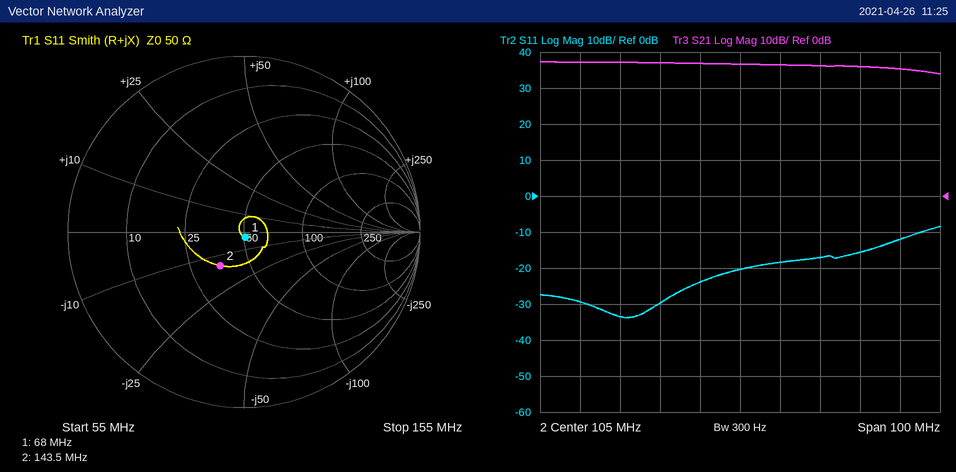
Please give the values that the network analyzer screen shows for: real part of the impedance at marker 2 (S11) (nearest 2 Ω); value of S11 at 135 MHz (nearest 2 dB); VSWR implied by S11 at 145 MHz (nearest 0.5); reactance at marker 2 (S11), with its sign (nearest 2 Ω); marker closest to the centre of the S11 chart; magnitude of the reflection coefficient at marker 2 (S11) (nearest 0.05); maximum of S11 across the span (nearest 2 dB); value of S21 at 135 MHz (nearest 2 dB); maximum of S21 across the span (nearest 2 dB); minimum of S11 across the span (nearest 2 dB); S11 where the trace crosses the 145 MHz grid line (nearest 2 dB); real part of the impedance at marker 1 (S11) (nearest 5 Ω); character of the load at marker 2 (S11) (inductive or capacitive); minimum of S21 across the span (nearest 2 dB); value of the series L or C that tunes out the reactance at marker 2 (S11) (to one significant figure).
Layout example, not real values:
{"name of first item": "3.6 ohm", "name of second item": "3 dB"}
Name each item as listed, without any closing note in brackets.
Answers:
{"real part of the impedance at marker 2 (S11)": "36 Ω", "value of S11 at 135 MHz": "-16 dB", "VSWR implied by S11 at 145 MHz": "1.5", "reactance at marker 2 (S11), with its sign": "-14 Ω", "marker closest to the centre of the S11 chart": "marker 1", "magnitude of the reflection coefficient at marker 2 (S11)": "0.25", "maximum of S11 across the span": "-8 dB", "value of S21 at 135 MHz": "36 dB", "maximum of S21 across the span": "38 dB", "minimum of S11 across the span": "-34 dB", "S11 where the trace crosses the 145 MHz grid line": "-12 dB", "real part of the impedance at marker 1 (S11)": "50 Ω", "character of the load at marker 2 (S11)": "capacitive", "minimum of S21 across the span": "34 dB", "value of the series L or C that tunes out the reactance at marker 2 (S11)": "20 nH"}
